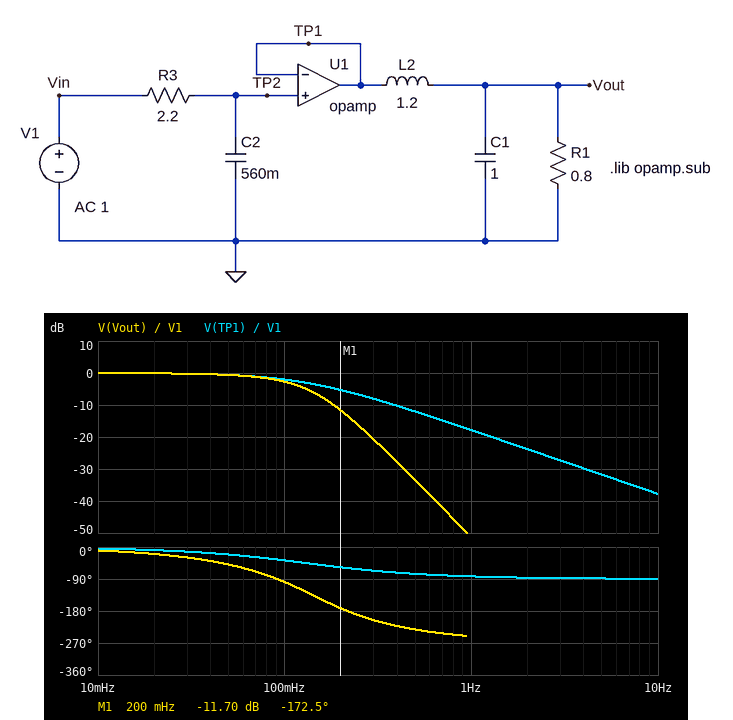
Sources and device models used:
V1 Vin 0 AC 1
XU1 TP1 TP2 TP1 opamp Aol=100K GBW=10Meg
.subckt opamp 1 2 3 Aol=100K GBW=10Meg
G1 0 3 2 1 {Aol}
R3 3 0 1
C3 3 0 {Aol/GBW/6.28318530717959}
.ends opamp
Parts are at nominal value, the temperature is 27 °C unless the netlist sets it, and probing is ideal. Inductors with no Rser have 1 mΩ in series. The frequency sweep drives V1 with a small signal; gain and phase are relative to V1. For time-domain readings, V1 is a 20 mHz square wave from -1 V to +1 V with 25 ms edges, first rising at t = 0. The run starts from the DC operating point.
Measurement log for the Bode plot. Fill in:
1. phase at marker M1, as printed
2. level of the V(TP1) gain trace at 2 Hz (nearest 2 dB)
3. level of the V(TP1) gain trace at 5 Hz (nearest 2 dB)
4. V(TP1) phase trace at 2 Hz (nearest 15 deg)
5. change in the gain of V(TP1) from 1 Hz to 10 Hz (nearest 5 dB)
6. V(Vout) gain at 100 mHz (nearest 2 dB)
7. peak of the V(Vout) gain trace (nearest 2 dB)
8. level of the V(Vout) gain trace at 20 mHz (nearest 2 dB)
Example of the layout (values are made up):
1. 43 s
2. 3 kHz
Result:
1. -172.5 deg
2. -24 dB
3. -32 dB
4. -90 deg
5. -20 dB
6. -2 dB
7. 0 dB
8. 0 dB
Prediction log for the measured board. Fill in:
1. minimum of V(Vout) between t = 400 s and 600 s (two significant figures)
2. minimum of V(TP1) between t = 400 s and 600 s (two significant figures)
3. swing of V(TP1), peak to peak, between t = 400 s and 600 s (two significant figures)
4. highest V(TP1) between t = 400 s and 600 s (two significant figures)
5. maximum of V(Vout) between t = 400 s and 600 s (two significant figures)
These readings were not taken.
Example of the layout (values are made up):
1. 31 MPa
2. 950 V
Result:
1. -1.0 V
2. -1.0 V
3. 2.0 V
4. 1.0 V
5. 1.0 V
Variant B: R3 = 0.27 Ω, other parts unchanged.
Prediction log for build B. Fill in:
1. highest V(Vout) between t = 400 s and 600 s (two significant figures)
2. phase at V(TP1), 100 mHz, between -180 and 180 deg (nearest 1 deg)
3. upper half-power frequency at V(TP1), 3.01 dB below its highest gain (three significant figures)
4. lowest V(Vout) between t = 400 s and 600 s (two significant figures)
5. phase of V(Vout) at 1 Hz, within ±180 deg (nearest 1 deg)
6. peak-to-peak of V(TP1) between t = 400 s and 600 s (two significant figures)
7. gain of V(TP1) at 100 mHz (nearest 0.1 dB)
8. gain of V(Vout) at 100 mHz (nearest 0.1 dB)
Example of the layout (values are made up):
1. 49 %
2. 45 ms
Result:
1. 1.1 V
2. -5 deg
3. 1.05 Hz
4. -1.1 V
5. 148 deg
6. 2.0 V
7. 0 dB
8. -0.7 dB
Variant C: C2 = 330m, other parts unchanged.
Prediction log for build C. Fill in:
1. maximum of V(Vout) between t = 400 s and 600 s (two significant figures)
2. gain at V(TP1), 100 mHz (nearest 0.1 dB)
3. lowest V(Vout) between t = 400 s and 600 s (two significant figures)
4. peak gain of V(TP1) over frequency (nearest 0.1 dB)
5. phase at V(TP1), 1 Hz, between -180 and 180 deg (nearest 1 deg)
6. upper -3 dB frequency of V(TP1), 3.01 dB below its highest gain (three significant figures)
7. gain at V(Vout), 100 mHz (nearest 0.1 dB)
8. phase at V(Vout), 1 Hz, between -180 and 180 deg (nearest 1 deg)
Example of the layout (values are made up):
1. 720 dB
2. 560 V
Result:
1. 1.1 V
2. -0.8 dB
3. -1.1 V
4. 0 dB
5. -78 deg
6. 219 mHz
7. -1.5 dB
8. 114 deg
